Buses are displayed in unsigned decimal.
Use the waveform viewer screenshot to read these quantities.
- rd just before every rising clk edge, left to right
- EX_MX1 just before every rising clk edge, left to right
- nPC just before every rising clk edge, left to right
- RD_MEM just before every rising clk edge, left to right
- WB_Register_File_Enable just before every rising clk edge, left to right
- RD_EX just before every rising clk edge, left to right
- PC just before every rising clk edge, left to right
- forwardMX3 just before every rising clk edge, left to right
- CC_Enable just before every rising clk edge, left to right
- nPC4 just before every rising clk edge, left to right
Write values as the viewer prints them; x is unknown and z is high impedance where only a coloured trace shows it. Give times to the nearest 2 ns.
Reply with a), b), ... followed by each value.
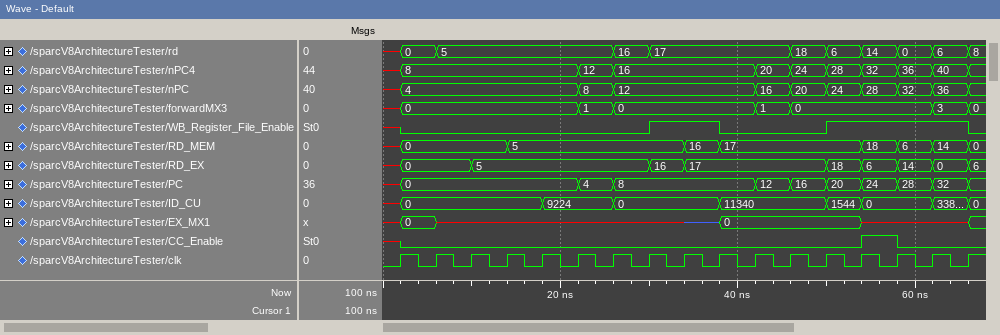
a) x, 0, 5, 5, 5, 5, 5, 16, 17, 17, 17, 17, 18, 6, 14, 0, 6
b) x, 0, x, x, x, x, x, x, x, z, 0, 0, 0, 0, x, x, x
c) x, 4, 4, 4, 4, 4, 8, 12, 12, 12, 12, 16, 20, 24, 28, 32, 36
d) x, 0, 0, 0, 5, 5, 5, 5, 5, 16, 17, 17, 17, 17, 18, 6, 14
e) x 0 0 0 0 0 0 0 1 1 0 0 0 1 1 1 1
f) x, 0, 0, 5, 5, 5, 5, 5, 16, 17, 17, 17, 17, 18, 6, 14, 0
g) x, 0, 0, 0, 0, 0, 4, 8, 8, 8, 8, 12, 16, 20, 24, 28, 32
h) x, 0, 0, 0, 0, 0, 1, 0, 0, 0, 0, 1, 0, 0, 0, 0, 3
i) x 0 0 0 0 0 0 0 0 0 0 0 0 0 1 0 0
j) x, 8, 8, 8, 8, 8, 12, 16, 16, 16, 16, 20, 24, 28, 32, 36, 40
